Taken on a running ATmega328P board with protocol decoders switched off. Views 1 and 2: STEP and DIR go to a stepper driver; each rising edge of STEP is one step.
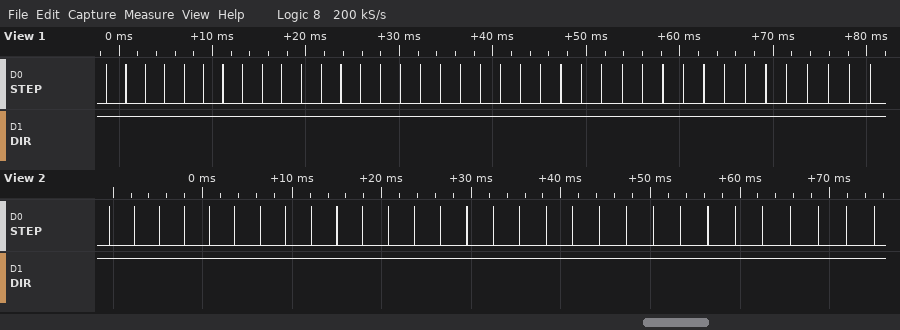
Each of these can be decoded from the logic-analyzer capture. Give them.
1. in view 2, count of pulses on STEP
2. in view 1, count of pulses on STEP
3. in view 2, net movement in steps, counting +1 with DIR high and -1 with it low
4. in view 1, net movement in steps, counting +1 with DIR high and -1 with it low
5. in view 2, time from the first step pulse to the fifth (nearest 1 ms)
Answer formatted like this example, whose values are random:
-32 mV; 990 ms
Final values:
30; 39; +30; +39; 11 ms
